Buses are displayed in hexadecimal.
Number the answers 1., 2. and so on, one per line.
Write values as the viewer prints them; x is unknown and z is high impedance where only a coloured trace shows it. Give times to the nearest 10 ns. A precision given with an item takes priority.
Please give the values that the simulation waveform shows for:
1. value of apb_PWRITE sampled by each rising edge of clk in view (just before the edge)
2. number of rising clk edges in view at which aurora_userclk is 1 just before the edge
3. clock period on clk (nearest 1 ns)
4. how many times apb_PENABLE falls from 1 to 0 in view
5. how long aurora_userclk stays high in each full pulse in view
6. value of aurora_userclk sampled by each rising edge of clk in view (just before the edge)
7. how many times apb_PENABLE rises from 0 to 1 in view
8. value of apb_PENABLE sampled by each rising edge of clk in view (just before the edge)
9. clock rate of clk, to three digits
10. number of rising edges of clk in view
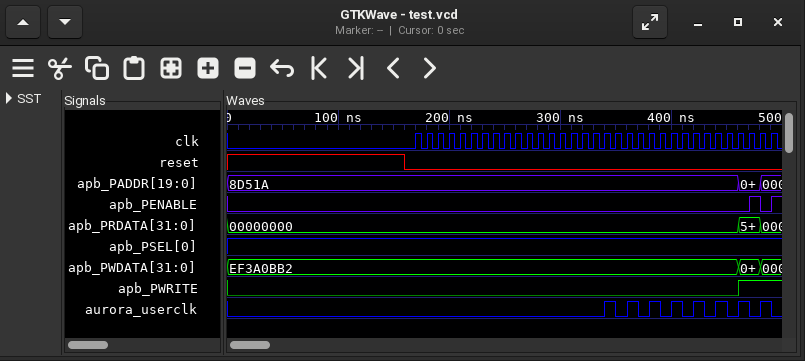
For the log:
1. 0 0 0 0 0 0 0 0 0 0 0 0 0 0 0 0 0 0 0 0 0 0 0 0 0 0 0 0 0 0 1 1 1
2. 8
3. 10 ns
4. 1
5. 10 ns, 10 ns, 10 ns, 10 ns, 10 ns, 10 ns, 10 ns, 10 ns
6. 0 0 0 0 0 0 0 0 0 0 0 0 0 0 0 0 0 0 1 0 1 0 1 0 1 0 1 0 1 0 1 0 1
7. 2
8. 0 0 0 0 0 0 0 0 0 0 0 0 0 0 0 0 0 0 0 0 0 0 0 0 0 0 0 0 0 0 0 1 0
9. 100 MHz
10. 33
